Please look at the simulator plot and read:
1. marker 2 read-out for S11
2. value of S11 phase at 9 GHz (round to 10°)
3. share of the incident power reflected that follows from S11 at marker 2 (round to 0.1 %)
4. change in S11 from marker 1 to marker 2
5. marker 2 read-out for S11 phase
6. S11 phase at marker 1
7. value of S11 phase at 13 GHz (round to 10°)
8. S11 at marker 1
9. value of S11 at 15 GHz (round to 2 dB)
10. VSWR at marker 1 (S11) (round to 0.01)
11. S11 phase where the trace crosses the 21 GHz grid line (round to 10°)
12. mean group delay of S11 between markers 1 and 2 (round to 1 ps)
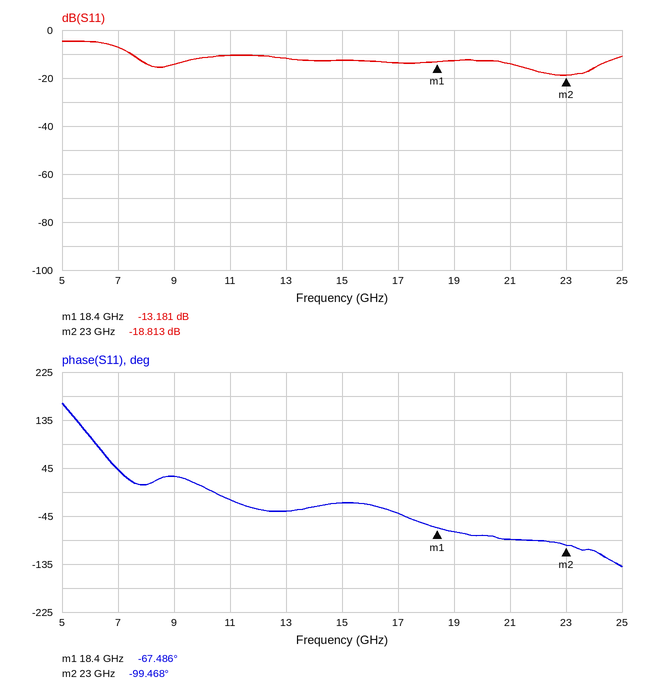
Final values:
-18.813 dB
30°
1.3 %
-5.632 dB
-99.468°
-67.486°
-40°
-13.181 dB
-12 dB
1.56
-90°
19 ps
